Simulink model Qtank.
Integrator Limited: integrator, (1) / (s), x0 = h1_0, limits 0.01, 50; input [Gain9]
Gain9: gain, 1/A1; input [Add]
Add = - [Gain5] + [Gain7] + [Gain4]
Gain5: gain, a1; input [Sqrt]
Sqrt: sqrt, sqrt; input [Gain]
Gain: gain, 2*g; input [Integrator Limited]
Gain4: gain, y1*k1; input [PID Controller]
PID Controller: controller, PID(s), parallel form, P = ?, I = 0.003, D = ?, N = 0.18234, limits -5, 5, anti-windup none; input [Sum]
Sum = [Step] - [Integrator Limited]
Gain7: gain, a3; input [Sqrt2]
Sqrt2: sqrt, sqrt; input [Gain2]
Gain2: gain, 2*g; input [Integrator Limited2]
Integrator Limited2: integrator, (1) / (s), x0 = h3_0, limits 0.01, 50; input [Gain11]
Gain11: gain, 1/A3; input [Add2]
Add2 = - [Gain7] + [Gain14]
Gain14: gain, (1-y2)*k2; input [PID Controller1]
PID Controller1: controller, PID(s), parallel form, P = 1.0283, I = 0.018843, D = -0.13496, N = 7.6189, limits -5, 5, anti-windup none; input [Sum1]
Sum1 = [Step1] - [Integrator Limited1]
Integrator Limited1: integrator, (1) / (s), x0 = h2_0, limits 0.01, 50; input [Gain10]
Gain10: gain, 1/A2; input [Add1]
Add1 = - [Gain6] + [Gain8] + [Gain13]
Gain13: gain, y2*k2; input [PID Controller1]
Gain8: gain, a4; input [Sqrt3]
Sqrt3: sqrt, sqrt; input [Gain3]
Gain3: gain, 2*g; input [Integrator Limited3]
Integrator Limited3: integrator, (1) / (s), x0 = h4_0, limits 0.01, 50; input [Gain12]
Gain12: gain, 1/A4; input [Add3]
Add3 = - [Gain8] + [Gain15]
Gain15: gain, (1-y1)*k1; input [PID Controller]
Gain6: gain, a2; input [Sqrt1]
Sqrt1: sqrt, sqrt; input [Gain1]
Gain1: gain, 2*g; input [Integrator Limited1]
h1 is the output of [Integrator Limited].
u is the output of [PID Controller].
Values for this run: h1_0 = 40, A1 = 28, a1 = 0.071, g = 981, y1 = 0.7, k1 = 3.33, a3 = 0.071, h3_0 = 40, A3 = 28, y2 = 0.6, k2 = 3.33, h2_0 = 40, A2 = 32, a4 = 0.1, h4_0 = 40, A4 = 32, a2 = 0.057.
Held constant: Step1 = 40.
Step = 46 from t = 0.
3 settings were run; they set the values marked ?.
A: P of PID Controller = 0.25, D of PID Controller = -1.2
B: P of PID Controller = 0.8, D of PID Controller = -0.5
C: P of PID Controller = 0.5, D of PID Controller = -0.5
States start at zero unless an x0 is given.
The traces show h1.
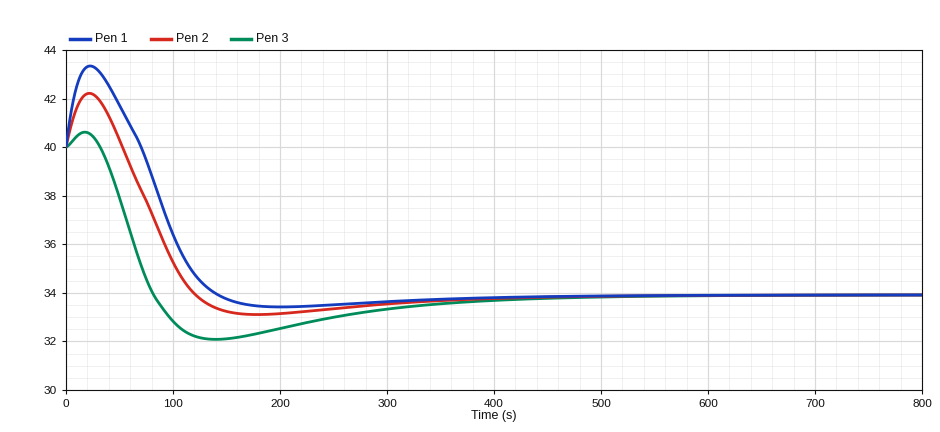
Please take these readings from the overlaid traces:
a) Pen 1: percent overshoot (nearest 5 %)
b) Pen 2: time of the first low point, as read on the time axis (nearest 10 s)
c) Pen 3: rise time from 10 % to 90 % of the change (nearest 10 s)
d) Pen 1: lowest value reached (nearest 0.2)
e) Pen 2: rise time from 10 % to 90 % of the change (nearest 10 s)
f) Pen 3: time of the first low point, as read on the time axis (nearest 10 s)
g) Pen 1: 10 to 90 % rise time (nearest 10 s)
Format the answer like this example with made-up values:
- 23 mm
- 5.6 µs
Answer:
- 10 %
- 180 s
- 40 s
- 33.4
- 50 s
- 140 s
- 50 s
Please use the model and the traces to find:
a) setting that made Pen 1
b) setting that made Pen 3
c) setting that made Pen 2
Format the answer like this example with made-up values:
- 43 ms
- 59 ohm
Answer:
- B
- A
- C
